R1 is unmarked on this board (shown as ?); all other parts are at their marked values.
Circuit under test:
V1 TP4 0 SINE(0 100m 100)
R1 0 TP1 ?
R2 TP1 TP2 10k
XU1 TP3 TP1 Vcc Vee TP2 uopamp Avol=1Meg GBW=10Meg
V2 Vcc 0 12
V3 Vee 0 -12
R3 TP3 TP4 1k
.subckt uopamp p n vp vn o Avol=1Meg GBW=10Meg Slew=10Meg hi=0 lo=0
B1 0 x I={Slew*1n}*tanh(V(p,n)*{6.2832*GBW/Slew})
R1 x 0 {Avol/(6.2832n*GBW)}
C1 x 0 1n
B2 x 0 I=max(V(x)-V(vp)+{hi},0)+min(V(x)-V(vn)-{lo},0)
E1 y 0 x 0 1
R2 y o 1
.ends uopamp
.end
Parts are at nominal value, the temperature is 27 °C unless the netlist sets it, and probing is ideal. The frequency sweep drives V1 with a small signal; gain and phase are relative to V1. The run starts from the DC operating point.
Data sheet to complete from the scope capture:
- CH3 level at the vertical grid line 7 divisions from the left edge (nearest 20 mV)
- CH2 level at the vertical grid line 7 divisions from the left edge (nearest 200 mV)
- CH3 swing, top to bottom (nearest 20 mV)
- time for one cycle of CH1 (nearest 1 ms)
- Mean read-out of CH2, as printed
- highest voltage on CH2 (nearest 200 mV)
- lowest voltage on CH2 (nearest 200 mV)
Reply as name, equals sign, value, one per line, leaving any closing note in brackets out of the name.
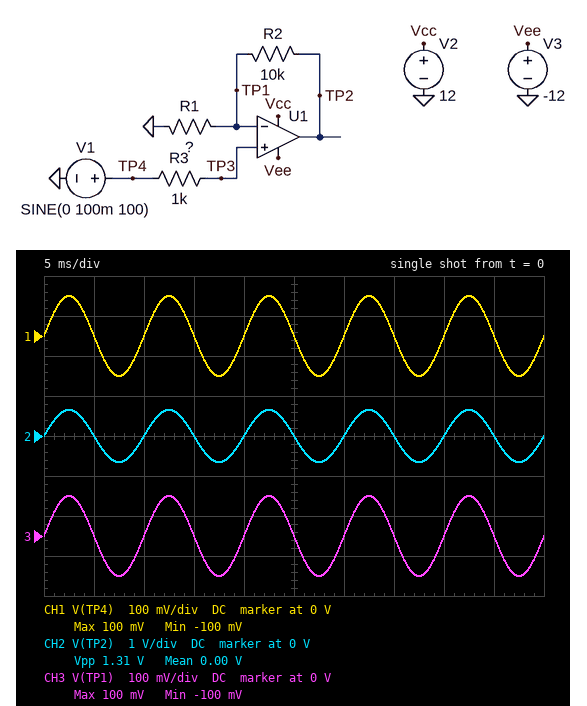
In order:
CH3 level at the vertical grid line 7 divisions from the left edge = 0 V
CH2 level at the vertical grid line 7 divisions from the left edge = 0 V
CH3 swing, top to bottom = 200 mV
time for one cycle of CH1 = 10 ms
Mean read-out of CH2, as printed = 0.00 V
highest voltage on CH2 = 600 mV
lowest voltage on CH2 = -600 mV
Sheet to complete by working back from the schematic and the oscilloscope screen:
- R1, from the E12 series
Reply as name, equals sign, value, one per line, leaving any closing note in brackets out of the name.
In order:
R1, from the E12 series = 1.8 kΩ
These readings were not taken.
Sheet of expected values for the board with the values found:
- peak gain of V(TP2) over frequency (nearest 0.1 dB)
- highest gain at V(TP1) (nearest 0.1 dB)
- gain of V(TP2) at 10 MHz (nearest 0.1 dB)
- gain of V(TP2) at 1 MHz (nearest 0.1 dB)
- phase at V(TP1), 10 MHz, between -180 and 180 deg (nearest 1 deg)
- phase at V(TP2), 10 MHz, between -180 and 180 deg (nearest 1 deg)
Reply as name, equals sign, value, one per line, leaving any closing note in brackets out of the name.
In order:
peak gain of V(TP2) over frequency = 16.3 dB
highest gain at V(TP1) = 0 dB
gain of V(TP2) at 10 MHz = -0.1 dB
gain of V(TP2) at 1 MHz = 14.8 dB
phase at V(TP1), 10 MHz, between -180 and 180 deg = -81 deg
phase at V(TP2), 10 MHz, between -180 and 180 deg = -81 deg
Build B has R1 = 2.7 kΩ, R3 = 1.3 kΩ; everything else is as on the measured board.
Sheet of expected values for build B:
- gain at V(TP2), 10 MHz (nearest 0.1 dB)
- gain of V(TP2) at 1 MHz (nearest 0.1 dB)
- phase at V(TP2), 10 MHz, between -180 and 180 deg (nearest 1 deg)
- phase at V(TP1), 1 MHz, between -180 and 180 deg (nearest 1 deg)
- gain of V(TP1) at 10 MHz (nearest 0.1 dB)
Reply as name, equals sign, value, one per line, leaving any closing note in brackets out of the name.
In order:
gain at V(TP2), 10 MHz = -0.2 dB
gain of V(TP2) at 1 MHz = 12.6 dB
phase at V(TP2), 10 MHz, between -180 and 180 deg = -78 deg
phase at V(TP1), 1 MHz, between -180 and 180 deg = -25 deg
gain of V(TP1) at 10 MHz = -13.6 dB
